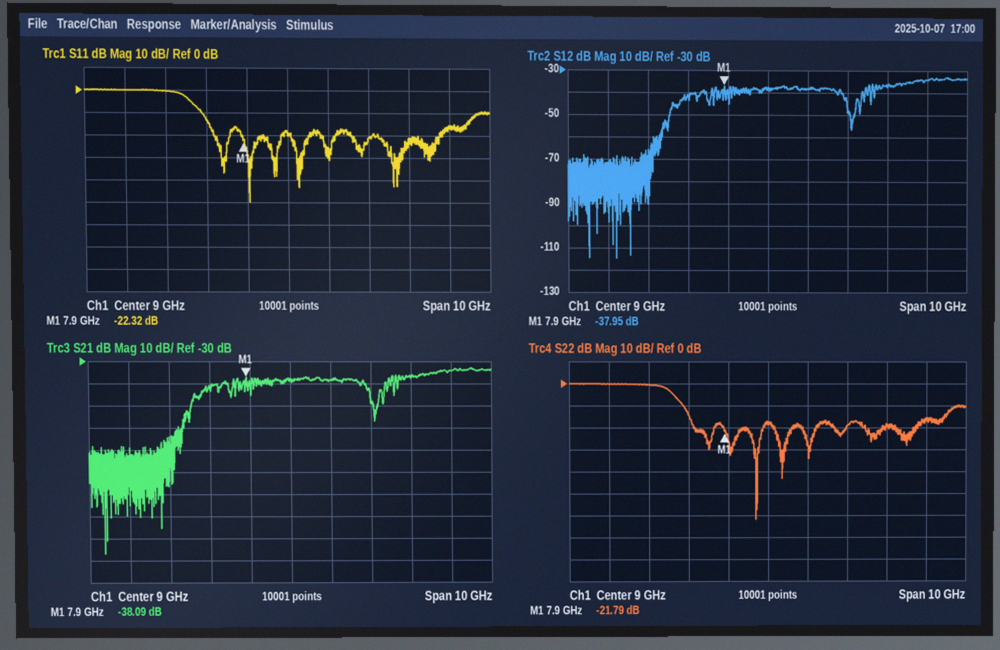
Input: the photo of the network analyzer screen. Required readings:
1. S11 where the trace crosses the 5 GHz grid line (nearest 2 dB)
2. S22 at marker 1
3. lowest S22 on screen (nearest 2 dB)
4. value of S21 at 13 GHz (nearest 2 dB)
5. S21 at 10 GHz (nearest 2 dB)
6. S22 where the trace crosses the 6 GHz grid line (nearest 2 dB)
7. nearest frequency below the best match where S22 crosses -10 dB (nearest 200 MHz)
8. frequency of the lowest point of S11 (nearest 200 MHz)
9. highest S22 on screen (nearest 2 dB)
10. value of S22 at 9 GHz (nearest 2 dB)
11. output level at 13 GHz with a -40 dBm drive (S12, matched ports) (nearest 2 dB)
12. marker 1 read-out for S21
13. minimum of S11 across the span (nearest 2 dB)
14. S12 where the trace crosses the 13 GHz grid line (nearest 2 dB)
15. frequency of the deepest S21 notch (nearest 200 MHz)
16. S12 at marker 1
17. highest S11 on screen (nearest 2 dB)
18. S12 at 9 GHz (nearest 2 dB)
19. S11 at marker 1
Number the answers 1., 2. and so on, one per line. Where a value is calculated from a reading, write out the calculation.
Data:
1. 0 dB
2. -21.79 dB
3. -62 dB
4. -34 dB
5. -38 dB
6. 0 dB
7. 6.8 GHz
8. 8.0 GHz
9. 0 dB
10. -18 dB
11. -40 dBm + (-34 dB) = -74 dBm
12. -38.09 dB
13. -50 dB
14. -34 dB
15. 4.4 GHz
16. -37.95 dB
17. 0 dB
18. -38 dB
19. -22.32 dB
